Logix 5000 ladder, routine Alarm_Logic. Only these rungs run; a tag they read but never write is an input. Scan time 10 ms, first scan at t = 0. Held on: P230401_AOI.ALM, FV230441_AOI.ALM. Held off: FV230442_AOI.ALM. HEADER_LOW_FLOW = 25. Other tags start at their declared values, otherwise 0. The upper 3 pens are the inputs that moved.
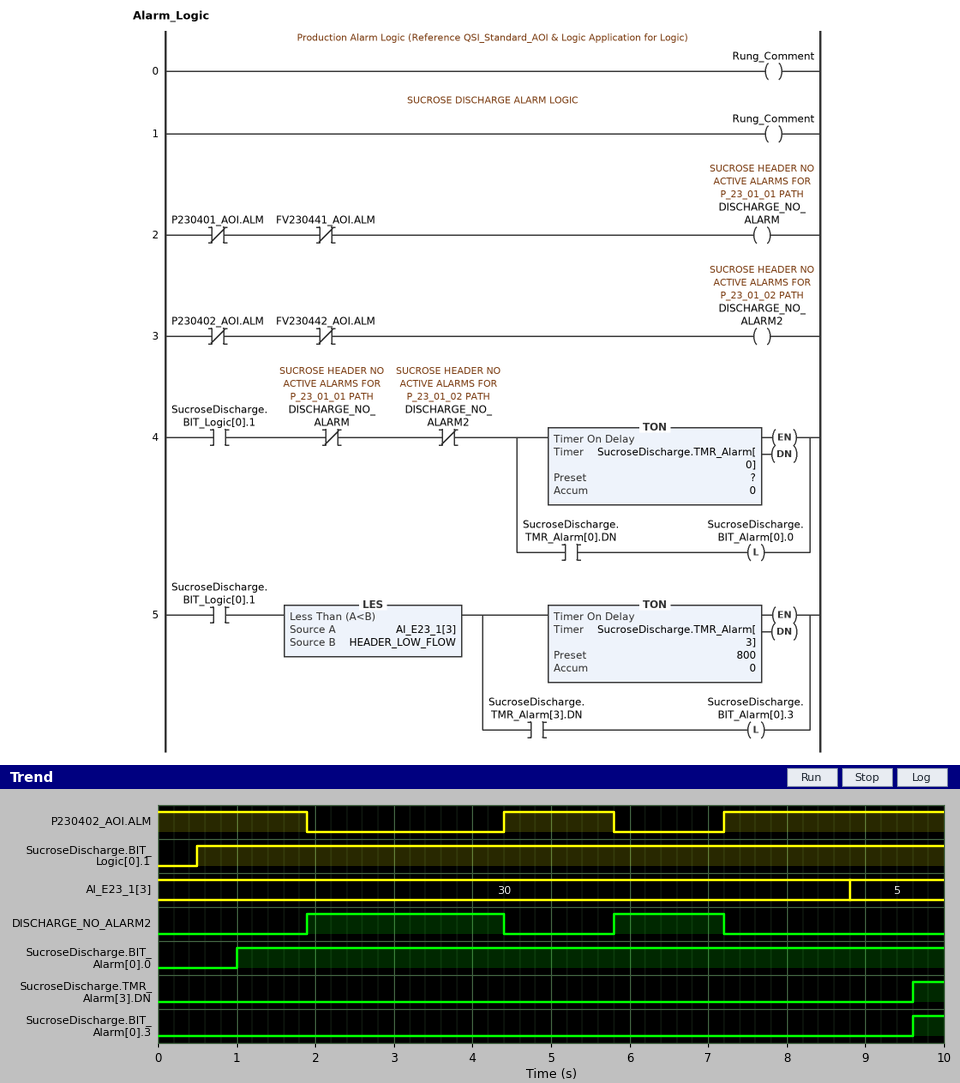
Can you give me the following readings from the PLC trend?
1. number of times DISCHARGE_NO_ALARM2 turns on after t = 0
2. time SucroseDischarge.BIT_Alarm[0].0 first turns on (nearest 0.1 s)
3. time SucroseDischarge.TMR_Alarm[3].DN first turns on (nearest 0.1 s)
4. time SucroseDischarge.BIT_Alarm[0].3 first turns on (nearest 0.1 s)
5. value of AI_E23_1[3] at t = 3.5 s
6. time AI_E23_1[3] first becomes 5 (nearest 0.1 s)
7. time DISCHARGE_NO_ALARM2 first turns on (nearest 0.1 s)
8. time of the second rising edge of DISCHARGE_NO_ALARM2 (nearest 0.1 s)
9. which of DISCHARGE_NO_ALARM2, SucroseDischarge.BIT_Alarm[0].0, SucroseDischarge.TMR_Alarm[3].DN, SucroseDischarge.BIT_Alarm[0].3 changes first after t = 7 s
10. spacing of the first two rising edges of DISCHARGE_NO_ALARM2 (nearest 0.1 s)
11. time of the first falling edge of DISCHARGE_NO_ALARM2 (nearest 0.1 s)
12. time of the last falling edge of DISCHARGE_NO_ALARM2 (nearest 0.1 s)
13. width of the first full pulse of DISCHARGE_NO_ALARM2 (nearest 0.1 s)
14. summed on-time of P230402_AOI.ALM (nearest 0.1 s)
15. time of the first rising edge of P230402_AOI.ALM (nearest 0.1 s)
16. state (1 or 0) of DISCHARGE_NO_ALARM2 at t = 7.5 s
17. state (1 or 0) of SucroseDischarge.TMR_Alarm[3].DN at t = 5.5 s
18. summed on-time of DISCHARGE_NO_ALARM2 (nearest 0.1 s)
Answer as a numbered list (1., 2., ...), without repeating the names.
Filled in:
1. 2
2. 1.0 s
3. 9.6 s
4. 9.6 s
5. 30
6. 8.8 s
7. 1.9 s
8. 5.8 s
9. DISCHARGE_NO_ALARM2
10. 3.9 s
11. 4.4 s
12. 7.2 s
13. 2.5 s
14. 6.1 s
15. 4.4 s
16. 0
17. 0
18. 3.9 s
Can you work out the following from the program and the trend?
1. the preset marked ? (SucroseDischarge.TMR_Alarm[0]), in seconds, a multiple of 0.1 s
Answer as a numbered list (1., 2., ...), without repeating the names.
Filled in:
1. 0.5 s
